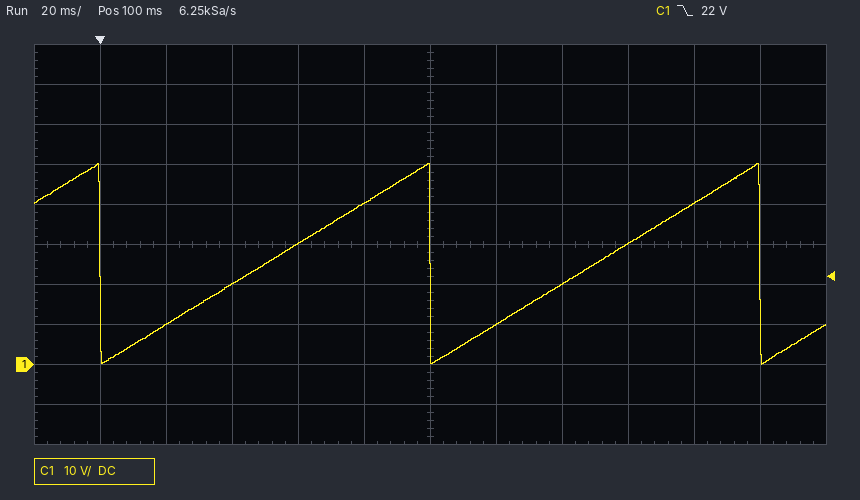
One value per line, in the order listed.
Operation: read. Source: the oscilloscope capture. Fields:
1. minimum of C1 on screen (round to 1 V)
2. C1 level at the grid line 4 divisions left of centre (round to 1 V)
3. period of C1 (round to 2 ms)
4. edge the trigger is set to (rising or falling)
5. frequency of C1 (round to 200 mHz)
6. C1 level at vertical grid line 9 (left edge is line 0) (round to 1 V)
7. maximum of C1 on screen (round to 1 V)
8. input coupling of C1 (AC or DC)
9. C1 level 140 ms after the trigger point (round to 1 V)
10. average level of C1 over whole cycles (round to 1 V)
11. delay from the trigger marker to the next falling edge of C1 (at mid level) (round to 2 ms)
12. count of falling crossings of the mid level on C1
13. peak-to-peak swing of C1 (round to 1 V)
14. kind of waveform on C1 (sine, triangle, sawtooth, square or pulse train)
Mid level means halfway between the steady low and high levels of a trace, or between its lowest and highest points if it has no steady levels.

0 V
10 V
100 ms
falling
10.0 Hz
30 V
50 V
DC
20 V
25 V
100 ms
3
50 V
sawtooth
